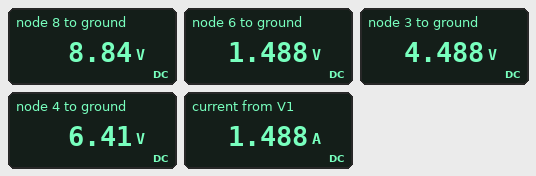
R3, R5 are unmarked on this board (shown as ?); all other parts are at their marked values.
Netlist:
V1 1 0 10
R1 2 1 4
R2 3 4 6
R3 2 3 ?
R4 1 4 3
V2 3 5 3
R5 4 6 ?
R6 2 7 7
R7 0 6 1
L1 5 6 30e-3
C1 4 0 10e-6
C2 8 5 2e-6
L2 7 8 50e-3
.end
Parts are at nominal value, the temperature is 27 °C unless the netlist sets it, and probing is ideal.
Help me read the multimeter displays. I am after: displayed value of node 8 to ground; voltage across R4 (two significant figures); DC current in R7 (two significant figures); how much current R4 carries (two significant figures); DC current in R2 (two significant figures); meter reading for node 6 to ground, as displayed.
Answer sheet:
8.84 V
3.6 V
1.5 A
1.2 A
320 mA
1.488 V
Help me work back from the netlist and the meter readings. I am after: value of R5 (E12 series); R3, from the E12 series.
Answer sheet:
5.6 Ω
15 Ω
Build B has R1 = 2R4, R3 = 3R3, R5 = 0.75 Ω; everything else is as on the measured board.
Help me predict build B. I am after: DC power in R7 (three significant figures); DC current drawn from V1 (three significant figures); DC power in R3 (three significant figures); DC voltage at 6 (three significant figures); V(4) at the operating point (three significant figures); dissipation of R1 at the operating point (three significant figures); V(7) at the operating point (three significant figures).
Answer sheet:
7.12 W
2.67 A
1.91 W
2.67 V
4.27 V
1.39 W
8.18 V
